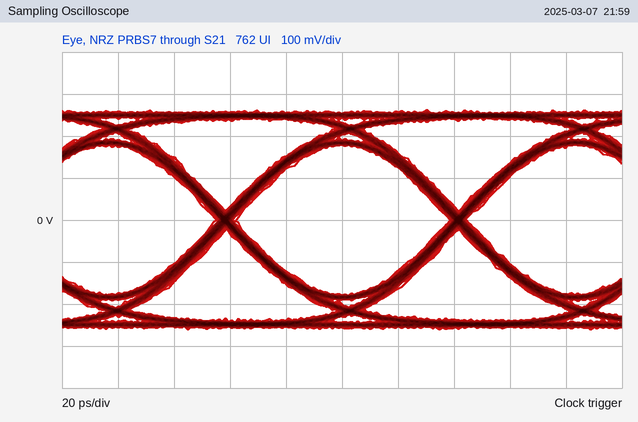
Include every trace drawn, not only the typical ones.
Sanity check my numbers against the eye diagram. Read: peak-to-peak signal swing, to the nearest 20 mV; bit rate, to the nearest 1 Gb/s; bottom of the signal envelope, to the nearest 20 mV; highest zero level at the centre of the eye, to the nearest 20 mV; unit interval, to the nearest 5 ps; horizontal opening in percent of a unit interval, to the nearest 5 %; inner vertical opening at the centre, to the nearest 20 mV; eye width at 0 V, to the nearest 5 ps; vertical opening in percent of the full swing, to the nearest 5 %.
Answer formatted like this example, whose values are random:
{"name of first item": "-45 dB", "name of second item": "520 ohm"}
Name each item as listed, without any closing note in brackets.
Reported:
{"peak-to-peak signal swing, to the nearest 20 mV": "520 mV", "bit rate, to the nearest 1 Gb/s": "12 Gb/s", "bottom of the signal envelope, to the nearest 20 mV": "-260 mV", "highest zero level at the centre of the eye, to the nearest 20 mV": "-180 mV", "unit interval, to the nearest 5 ps": "85 ps", "horizontal opening in percent of a unit interval, to the nearest 5 %": "90 %", "inner vertical opening at the centre, to the nearest 20 mV": "360 mV", "eye width at 0 V, to the nearest 5 ps": "75 ps", "vertical opening in percent of the full swing, to the nearest 5 %": "70 %"}
